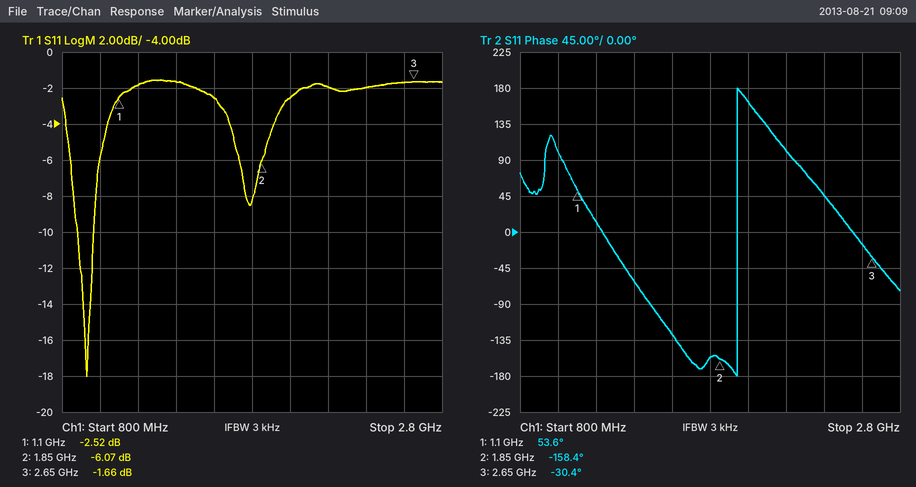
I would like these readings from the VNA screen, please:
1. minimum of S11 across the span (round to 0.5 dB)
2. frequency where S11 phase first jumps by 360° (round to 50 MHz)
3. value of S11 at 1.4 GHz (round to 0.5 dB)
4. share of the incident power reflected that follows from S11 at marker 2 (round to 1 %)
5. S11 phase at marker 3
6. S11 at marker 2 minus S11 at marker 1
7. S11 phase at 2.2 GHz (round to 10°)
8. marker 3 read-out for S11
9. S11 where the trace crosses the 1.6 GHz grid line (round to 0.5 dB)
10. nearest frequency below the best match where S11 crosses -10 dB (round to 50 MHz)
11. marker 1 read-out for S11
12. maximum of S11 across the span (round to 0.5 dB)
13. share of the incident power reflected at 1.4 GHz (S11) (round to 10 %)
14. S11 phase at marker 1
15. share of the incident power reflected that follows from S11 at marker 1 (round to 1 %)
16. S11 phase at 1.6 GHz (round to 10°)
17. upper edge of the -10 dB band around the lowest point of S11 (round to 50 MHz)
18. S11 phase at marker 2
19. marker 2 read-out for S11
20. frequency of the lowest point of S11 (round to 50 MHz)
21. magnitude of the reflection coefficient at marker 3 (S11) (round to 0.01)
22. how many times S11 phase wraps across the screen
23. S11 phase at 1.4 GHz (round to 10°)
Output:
-18.0 dB
1.95 GHz
-1.5 dB
25 %
-30.4°
-3.55 dB
100°
-1.66 dB
-2.5 dB
900 MHz
-2.52 dB
-1.5 dB
70 %
53.6°
56 %
-130°
950 MHz
-158.4°
-6.07 dB
950 MHz
0.83
1
-60°
